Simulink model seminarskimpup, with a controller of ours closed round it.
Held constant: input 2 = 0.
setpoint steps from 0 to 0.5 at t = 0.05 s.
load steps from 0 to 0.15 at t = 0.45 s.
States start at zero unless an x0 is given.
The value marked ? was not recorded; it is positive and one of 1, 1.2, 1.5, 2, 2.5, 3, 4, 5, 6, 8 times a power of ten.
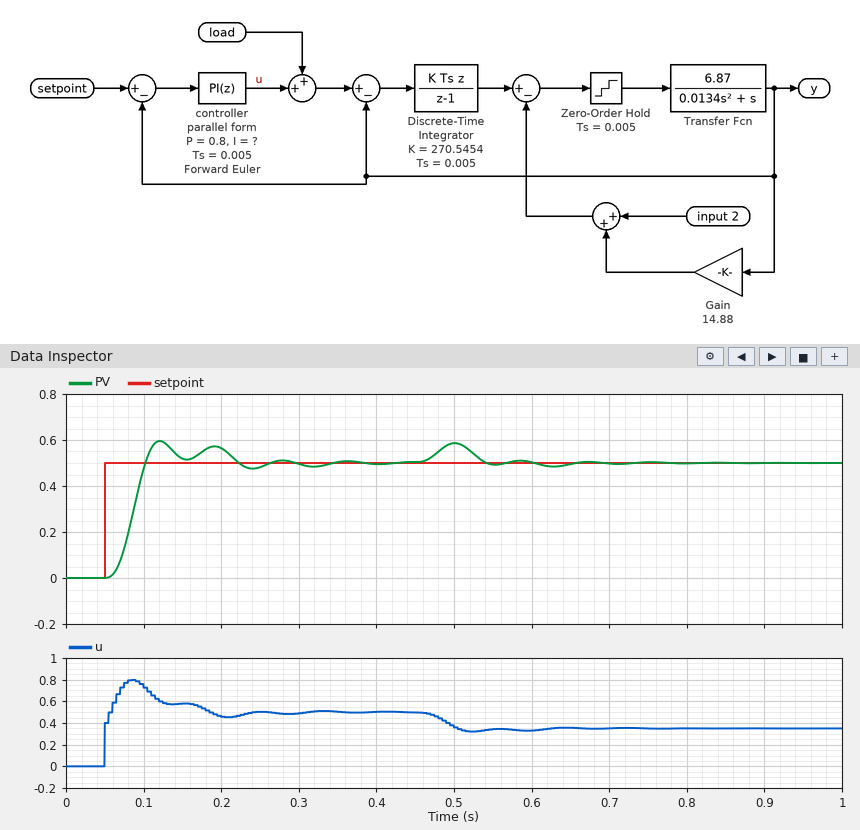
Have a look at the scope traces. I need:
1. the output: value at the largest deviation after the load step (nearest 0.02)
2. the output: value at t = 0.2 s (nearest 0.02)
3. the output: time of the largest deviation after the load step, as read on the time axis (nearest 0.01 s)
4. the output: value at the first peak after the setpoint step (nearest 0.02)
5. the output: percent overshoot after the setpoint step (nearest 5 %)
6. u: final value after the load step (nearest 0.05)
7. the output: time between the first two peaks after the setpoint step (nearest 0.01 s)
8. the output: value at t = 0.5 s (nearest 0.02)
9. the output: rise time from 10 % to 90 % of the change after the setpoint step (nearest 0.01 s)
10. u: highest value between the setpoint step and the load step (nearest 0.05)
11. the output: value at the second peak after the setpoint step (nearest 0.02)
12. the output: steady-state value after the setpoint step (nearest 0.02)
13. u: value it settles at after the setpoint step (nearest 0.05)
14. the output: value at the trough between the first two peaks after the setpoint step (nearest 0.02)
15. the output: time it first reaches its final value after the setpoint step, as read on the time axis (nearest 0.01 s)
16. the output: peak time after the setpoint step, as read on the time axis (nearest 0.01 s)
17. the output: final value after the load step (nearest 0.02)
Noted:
0.58
0.56
0.50 s
0.60
20 %
0.35
0.07 s
0.58
0.03 s
0.80
0.58
0.50
0.50
0.52
0.10 s
0.12 s
0.50
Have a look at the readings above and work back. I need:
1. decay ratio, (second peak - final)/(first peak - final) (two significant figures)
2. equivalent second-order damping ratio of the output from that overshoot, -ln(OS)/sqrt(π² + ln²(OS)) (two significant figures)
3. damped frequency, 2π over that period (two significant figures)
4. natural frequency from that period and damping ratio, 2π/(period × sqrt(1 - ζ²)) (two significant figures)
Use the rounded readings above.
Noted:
0.80
0.46
90 rad/s
100 rad/s
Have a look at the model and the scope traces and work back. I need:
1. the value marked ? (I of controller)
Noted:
40
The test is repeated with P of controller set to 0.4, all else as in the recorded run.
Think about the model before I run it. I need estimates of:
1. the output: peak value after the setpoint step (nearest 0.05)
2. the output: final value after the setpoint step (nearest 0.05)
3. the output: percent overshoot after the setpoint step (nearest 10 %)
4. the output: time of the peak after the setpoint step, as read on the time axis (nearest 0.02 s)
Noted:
0.65
0.50
30 %
0.14 s
